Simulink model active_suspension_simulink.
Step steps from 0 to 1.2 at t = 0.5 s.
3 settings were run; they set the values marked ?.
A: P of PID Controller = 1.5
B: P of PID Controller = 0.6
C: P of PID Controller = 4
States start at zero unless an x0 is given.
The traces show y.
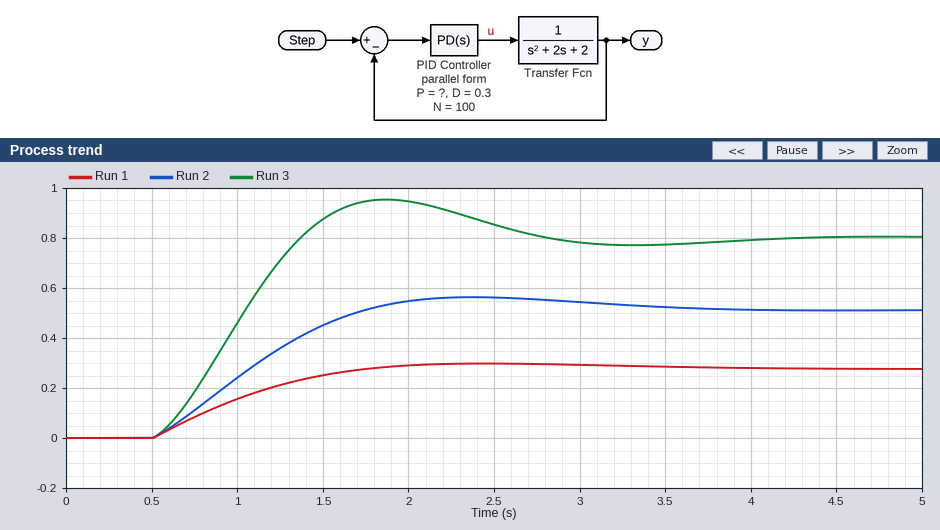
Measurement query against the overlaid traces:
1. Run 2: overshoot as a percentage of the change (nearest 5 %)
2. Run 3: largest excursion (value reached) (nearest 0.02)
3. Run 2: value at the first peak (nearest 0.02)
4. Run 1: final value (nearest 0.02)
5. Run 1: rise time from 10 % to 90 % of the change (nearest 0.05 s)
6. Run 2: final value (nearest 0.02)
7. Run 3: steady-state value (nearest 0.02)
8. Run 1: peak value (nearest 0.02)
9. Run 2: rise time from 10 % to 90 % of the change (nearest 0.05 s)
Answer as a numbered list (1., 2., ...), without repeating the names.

1. 10 %
2. 0.96
3. 0.56
4. 0.28
5. 0.90 s
6. 0.52
7. 0.80
8. 0.30
9. 0.90 s
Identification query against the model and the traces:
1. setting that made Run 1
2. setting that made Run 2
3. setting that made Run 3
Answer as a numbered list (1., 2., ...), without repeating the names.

1. B
2. A
3. C
